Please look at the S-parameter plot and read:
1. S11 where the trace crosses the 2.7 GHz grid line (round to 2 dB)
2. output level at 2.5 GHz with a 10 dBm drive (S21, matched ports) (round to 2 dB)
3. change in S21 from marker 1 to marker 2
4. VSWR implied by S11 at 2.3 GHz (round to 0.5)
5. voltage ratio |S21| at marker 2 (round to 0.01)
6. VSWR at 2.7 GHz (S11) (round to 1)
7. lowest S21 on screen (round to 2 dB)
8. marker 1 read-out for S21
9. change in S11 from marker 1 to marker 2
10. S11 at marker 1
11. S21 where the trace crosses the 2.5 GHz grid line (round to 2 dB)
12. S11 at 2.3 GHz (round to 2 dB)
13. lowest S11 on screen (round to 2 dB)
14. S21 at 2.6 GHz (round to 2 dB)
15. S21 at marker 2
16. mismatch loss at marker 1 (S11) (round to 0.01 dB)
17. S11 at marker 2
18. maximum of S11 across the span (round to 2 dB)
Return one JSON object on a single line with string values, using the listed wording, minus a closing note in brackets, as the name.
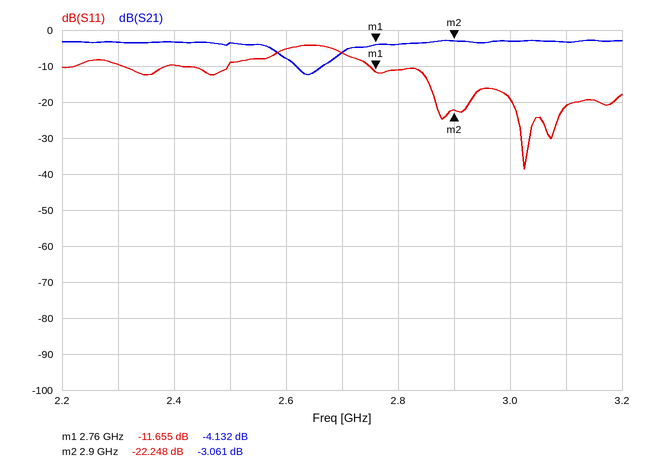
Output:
{"S11 where the trace crosses the 2.7 GHz grid line": "-6 dB", "output level at 2.5 GHz with a 10 dBm drive (S21, matched ports)": "6 dBm", "change in S21 from marker 1 to marker 2": "1.071 dB", "VSWR implied by S11 at 2.3 GHz": "2.0", "voltage ratio |S21| at marker 2": "0.70", "VSWR at 2.7 GHz (S11)": "3", "lowest S21 on screen": "-12 dB", "marker 1 read-out for S21": "-4.132 dB", "change in S11 from marker 1 to marker 2": "-10.593 dB", "S11 at marker 1": "-11.655 dB", "S21 where the trace crosses the 2.5 GHz grid line": "-4 dB", "S11 at 2.3 GHz": "-10 dB", "lowest S11 on screen": "-38 dB", "S21 at 2.6 GHz": "-8 dB", "S21 at marker 2": "-3.061 dB", "mismatch loss at marker 1 (S11)": "0.31 dB", "S11 at marker 2": "-22.248 dB", "maximum of S11 across the span": "-4 dB"}
